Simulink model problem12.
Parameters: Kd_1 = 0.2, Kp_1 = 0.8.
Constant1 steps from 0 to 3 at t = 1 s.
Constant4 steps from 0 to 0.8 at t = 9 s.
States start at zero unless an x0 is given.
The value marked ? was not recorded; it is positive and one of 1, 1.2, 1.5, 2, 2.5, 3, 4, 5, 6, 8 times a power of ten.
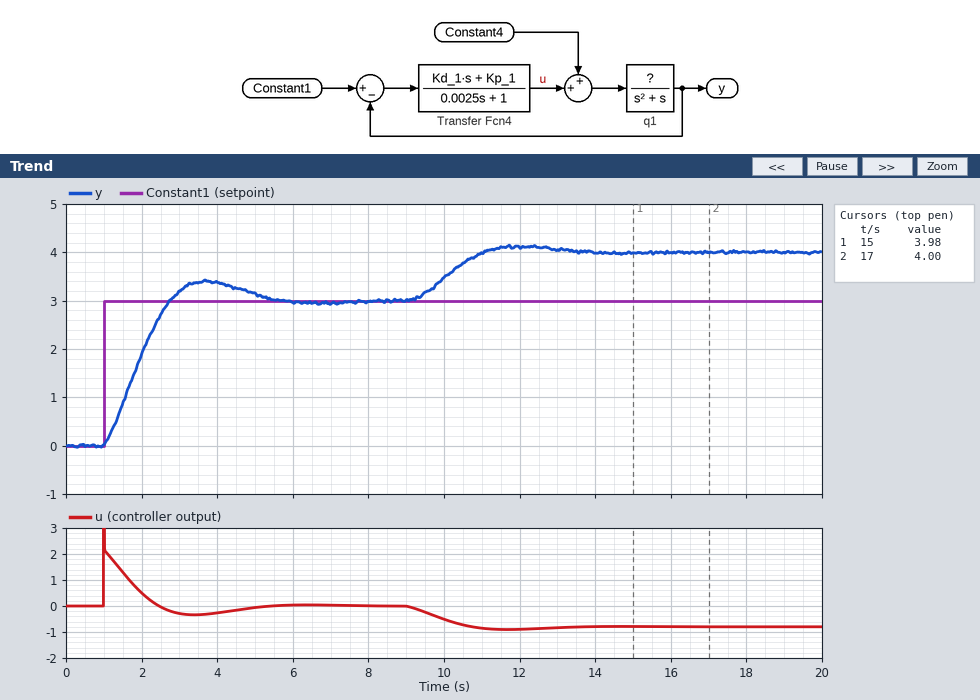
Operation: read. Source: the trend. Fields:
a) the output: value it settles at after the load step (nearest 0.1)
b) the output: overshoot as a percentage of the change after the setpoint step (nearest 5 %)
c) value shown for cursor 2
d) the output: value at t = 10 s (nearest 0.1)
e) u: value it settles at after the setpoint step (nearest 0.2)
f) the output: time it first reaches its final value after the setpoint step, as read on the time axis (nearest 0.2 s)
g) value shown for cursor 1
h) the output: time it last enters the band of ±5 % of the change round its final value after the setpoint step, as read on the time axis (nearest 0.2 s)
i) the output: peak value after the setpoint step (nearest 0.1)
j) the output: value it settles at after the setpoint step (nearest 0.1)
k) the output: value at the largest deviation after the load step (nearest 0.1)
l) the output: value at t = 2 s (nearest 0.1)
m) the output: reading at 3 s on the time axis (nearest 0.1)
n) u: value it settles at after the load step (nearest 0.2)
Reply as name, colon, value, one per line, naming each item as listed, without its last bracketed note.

the output: value it settles at after the load step: 4.0
the output: overshoot as a percentage of the change after the setpoint step: 15 %
value shown for cursor 2: 4.00
the output: value at t = 10 s: 3.5
u: value it settles at after the setpoint step: 0.0
the output: time it first reaches its final value after the setpoint step, as read on the time axis: 2.8 s
value shown for cursor 1: 3.98
the output: time it last enters the band of ±5 % of the change round its final value after the setpoint step, as read on the time axis: 5.0 s
the output: peak value after the setpoint step: 3.4
the output: value it settles at after the setpoint step: 3.0
the output: value at the largest deviation after the load step: 4.1
the output: value at t = 2 s: 1.9
the output: reading at 3 s on the time axis: 3.2
u: value it settles at after the load step: -0.8
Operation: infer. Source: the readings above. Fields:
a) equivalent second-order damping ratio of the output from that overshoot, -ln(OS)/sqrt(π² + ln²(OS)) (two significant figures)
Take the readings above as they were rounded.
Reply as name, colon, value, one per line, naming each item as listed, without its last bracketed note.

equivalent second-order damping ratio of the output from that overshoot, -ln(OS)/sqrt(π² + ln²(OS)): 0.52
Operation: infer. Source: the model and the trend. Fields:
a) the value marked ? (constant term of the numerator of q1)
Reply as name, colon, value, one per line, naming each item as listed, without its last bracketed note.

the value marked ?: 2
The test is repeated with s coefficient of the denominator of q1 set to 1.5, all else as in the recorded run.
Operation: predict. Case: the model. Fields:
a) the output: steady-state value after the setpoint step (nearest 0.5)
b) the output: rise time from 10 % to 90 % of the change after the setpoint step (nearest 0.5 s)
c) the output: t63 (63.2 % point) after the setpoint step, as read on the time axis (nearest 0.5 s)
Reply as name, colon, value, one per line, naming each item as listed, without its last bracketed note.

the output: steady-state value after the setpoint step: 3.0
the output: rise time from 10 % to 90 % of the change after the setpoint step: 1.5 s
the output: t63 (63.2 % point) after the setpoint step, as read on the time axis: 2.0 s
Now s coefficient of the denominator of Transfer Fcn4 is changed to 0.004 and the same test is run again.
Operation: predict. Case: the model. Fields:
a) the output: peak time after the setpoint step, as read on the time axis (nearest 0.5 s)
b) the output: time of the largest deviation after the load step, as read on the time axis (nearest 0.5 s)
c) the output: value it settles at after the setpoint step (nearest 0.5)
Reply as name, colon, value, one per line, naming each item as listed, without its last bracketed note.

the output: peak time after the setpoint step, as read on the time axis: 3.5 s
the output: time of the largest deviation after the load step, as read on the time axis: 12.0 s
the output: value it settles at after the setpoint step: 3.0
